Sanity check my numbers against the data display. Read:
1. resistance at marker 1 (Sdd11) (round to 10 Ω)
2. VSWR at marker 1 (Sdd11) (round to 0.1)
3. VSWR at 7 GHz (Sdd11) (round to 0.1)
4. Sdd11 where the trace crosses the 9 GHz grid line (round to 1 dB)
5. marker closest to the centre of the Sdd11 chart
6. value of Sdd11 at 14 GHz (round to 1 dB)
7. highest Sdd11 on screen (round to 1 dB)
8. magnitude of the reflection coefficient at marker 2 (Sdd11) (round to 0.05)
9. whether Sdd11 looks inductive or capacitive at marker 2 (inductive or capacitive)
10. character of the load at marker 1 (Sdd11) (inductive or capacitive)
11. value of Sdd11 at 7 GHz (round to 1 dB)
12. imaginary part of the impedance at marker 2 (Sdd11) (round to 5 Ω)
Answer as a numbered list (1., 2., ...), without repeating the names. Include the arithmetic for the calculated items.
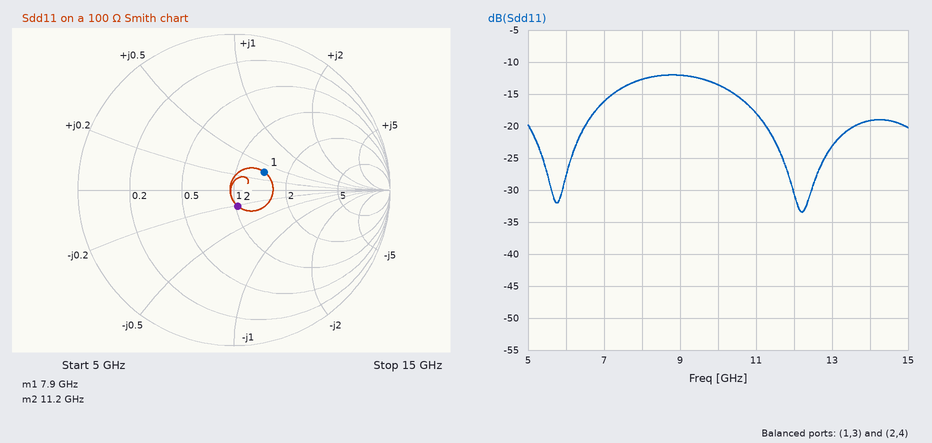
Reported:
1. 140 Ω
2. 1.6
3. |Γ| = 10^(-16/20) = 0.1585; VSWR = (1 + 0.1585)/(1 − 0.1585) ≈ 1.4
4. -12 dB
5. marker 2
6. -19 dB
7. -12 dB
8. 0.10
9. capacitive
10. inductive
11. -16 dB
12. -20 Ω
